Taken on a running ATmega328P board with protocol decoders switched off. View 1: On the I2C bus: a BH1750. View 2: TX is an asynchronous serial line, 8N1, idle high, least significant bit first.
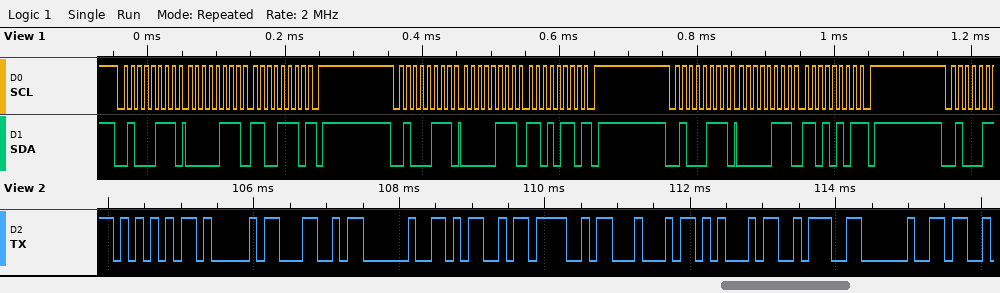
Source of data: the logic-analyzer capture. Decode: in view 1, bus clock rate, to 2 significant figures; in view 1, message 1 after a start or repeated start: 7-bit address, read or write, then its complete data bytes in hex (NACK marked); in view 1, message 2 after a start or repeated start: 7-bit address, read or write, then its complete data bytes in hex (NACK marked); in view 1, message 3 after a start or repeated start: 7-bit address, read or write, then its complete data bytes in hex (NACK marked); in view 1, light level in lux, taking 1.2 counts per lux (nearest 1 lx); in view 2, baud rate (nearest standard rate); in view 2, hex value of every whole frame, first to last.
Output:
100 kHz
0x23 read: 07 CE NACK
0x23 read: 07 D6 NACK
0x23 read: 07 D5 NACK
1665 lx
9600 baud
55 41 4C 20 4D 4F 44 45 3A 20
